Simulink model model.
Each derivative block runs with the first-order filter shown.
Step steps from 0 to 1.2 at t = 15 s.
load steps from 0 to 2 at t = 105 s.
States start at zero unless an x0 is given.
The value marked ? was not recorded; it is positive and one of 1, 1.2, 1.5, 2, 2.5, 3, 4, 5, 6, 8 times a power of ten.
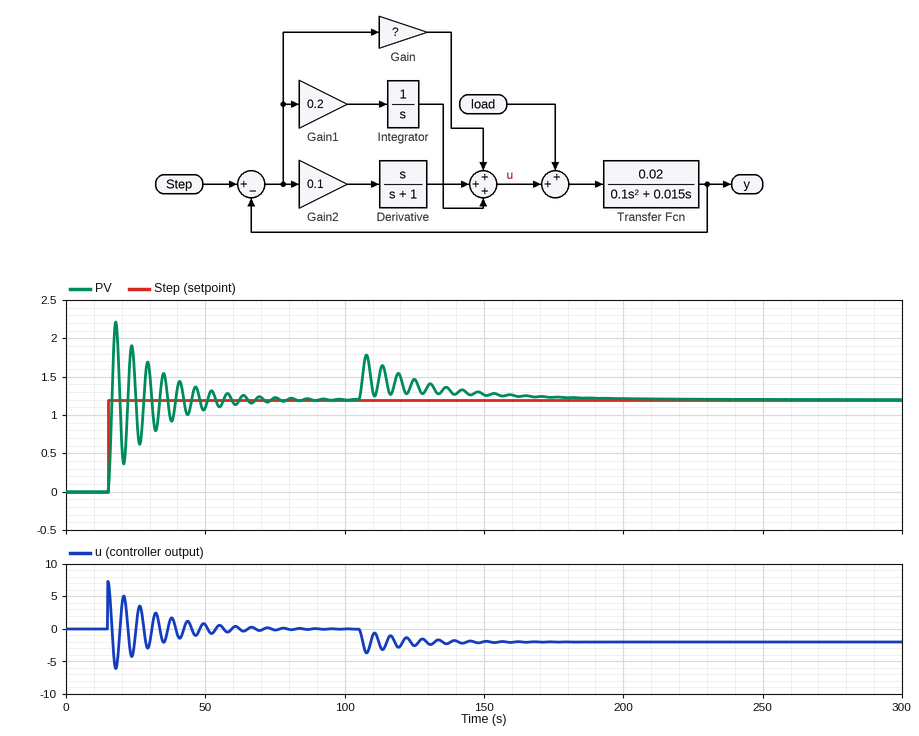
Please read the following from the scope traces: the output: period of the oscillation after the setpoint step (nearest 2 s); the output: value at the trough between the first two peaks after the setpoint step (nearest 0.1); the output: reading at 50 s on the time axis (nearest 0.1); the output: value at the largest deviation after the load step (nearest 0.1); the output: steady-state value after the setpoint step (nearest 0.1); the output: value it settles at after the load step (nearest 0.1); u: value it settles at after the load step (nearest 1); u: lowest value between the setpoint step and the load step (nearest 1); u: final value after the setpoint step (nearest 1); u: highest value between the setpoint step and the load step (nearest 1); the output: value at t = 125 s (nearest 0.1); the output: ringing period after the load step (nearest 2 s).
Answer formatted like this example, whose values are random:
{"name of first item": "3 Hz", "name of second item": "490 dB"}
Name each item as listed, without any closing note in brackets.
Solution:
{"the output: period of the oscillation after the setpoint step": "6 s", "the output: value at the trough between the first two peaks after the setpoint step": "0.4", "the output: reading at 50 s on the time axis": "1.1", "the output: value at the largest deviation after the load step": "1.8", "the output: steady-state value after the setpoint step": "1.2", "the output: value it settles at after the load step": "1.2", "u: value it settles at after the load step": "-2", "u: lowest value between the setpoint step and the load step": "-6", "u: final value after the setpoint step": "0", "u: highest value between the setpoint step and the load step": "7", "the output: value at t = 125 s": "1.5", "the output: ringing period after the load step": "6 s"}
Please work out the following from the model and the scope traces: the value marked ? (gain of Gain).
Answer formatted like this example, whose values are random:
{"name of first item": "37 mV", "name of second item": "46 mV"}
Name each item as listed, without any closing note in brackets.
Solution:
{"the value marked ?": "6"}
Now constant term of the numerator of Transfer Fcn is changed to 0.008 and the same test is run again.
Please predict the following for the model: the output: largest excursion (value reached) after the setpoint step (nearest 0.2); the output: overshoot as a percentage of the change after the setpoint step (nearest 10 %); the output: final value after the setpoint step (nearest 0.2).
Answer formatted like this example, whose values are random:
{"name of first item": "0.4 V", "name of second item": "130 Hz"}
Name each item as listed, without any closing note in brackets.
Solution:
{"the output: largest excursion (value reached) after the setpoint step": "2.2", "the output: overshoot as a percentage of the change after the setpoint step": "80 %", "the output: final value after the setpoint step": "1.2"}
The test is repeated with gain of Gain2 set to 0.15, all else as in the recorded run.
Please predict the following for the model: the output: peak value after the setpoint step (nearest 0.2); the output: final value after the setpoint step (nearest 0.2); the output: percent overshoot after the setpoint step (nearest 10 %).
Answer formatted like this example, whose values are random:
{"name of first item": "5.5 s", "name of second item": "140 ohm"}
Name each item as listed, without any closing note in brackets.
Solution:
{"the output: peak value after the setpoint step": "2.2", "the output: final value after the setpoint step": "1.2", "the output: percent overshoot after the setpoint step": "80 %"}
